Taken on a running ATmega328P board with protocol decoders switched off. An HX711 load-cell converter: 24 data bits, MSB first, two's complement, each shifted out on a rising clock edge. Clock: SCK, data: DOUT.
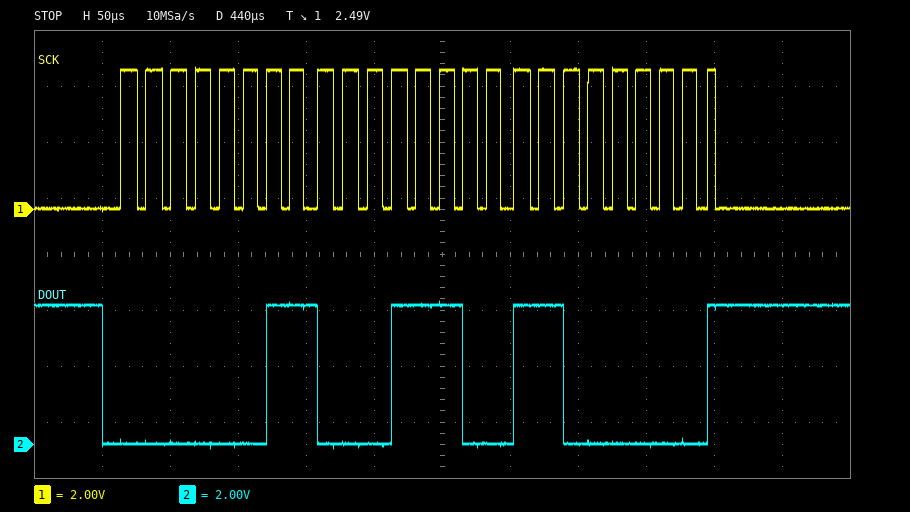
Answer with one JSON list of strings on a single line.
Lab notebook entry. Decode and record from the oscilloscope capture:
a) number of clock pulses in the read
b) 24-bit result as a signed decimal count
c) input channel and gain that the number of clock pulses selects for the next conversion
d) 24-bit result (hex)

["25", "203968", "channel A, gain 128", "0x031CC0"]
